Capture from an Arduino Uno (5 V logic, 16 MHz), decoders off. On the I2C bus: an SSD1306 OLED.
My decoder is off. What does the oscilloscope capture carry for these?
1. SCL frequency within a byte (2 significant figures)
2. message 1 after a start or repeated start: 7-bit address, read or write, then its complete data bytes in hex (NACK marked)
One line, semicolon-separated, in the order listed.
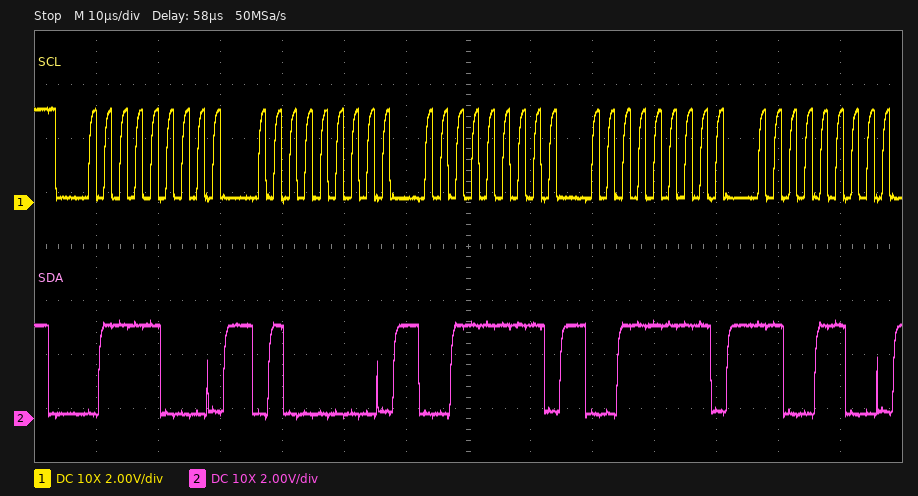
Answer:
400 kHz; 0x3C write: 40 3F 3F CC
